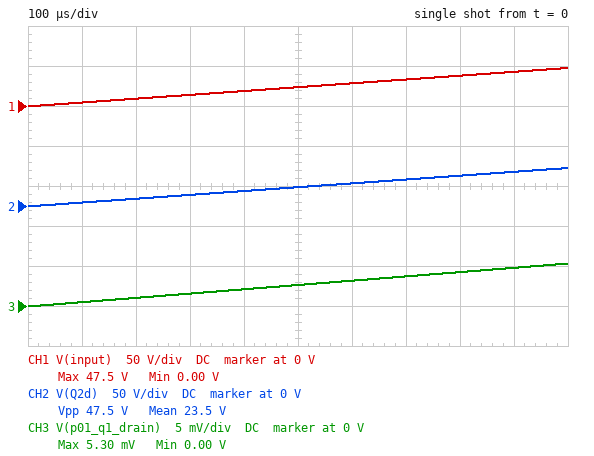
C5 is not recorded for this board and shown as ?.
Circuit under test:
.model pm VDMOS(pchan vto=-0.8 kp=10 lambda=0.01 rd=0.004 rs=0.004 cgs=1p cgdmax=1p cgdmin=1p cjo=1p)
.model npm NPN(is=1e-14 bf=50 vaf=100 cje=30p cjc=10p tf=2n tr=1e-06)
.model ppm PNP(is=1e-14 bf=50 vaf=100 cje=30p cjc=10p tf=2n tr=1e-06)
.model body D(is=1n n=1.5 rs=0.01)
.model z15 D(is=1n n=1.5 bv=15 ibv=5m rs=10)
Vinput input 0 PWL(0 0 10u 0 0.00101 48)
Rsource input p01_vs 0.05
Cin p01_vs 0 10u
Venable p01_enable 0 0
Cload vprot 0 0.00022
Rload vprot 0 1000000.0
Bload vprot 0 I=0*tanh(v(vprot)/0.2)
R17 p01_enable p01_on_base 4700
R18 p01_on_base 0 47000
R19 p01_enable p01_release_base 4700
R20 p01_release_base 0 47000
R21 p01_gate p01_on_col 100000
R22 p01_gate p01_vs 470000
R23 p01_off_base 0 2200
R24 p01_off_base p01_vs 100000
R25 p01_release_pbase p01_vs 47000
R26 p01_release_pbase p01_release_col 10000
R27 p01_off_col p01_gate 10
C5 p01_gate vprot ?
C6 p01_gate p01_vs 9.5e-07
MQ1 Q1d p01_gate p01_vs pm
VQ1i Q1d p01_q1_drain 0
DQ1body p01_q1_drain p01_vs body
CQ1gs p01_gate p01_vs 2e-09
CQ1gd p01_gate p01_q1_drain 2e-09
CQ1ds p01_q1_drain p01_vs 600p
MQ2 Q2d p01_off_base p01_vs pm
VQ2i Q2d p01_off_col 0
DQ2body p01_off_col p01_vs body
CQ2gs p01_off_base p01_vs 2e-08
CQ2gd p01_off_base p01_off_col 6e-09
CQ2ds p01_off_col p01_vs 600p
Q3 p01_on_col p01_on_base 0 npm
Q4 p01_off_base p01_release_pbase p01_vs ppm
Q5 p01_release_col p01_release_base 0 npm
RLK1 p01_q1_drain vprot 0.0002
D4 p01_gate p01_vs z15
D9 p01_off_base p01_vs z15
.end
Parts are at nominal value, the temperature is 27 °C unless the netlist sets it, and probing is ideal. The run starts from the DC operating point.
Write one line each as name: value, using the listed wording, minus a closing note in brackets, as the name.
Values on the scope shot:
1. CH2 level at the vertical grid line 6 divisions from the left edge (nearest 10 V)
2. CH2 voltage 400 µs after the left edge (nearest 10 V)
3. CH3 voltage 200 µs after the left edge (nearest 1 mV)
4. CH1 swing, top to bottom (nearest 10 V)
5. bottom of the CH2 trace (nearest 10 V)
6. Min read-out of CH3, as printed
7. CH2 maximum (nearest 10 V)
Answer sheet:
CH2 level at the vertical grid line 6 divisions from the left edge: 30 V
CH2 voltage 400 µs after the left edge: 20 V
CH3 voltage 200 µs after the left edge: 1 mV
CH1 swing, top to bottom: 50 V
bottom of the CH2 trace: 0 V
Min read-out of CH3, as printed: 0.00 V
CH2 maximum: 50 V
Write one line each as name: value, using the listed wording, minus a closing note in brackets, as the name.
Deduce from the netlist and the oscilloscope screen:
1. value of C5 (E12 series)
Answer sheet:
value of C5: 22 nF
